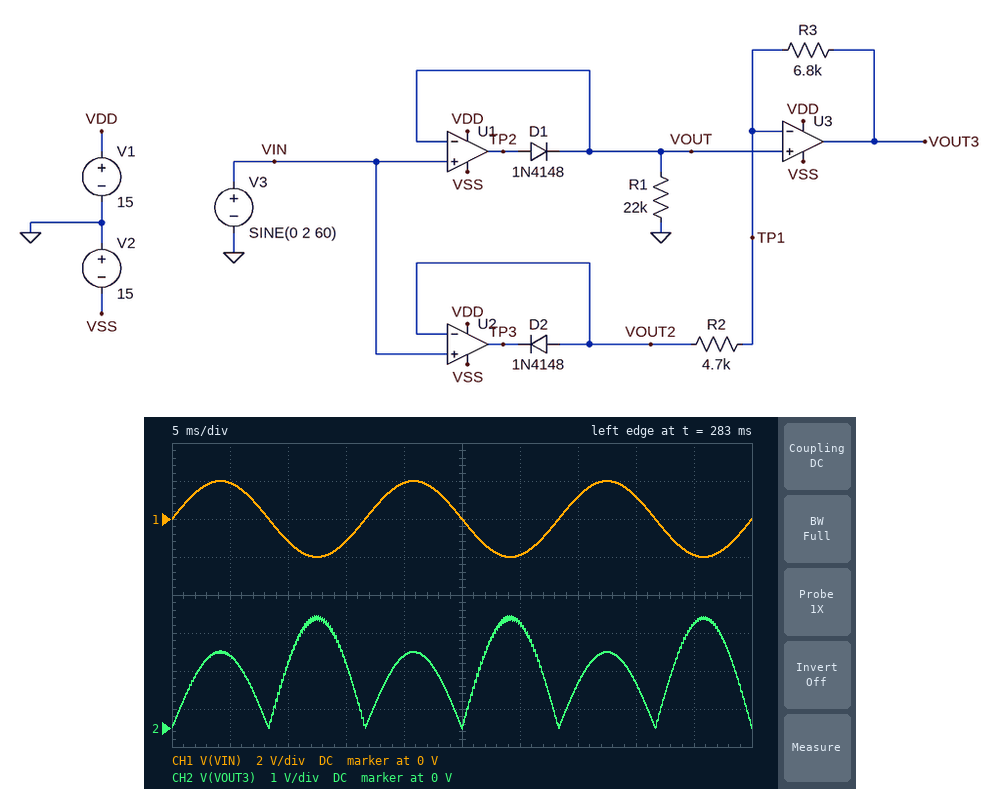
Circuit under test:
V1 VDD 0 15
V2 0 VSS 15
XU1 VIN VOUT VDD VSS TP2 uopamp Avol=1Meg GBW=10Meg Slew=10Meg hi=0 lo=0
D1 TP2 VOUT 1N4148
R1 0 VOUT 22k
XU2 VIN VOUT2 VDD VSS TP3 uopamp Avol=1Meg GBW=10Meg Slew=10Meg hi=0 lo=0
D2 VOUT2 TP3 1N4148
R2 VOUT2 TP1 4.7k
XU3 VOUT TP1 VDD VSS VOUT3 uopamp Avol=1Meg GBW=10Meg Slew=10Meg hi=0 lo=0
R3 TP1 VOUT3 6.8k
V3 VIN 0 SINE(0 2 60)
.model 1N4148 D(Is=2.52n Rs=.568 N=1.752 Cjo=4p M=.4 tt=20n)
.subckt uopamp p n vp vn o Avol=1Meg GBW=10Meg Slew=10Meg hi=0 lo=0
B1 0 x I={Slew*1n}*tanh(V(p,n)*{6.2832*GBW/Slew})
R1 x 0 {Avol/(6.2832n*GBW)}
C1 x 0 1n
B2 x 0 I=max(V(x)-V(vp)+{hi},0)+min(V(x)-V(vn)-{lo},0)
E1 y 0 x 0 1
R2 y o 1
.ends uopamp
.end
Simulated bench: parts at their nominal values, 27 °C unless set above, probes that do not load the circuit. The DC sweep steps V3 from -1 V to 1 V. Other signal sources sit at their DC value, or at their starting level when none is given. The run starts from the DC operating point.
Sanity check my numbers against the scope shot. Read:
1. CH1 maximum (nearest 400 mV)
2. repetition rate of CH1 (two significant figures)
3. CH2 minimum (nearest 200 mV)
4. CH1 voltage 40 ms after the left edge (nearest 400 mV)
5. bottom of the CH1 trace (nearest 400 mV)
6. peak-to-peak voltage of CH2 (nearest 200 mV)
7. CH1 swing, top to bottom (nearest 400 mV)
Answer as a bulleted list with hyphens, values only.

- 2.0 V
- 60 Hz
- 0 V
- 1.2 V
- -2.0 V
- 3.0 V
- 4.0 V
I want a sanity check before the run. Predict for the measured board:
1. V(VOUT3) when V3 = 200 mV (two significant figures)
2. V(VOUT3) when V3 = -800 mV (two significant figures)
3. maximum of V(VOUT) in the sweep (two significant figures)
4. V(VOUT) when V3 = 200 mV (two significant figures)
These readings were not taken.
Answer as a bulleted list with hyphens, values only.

- 200 mV
- 1.2 V
- 1.0 V
- 200 mV
